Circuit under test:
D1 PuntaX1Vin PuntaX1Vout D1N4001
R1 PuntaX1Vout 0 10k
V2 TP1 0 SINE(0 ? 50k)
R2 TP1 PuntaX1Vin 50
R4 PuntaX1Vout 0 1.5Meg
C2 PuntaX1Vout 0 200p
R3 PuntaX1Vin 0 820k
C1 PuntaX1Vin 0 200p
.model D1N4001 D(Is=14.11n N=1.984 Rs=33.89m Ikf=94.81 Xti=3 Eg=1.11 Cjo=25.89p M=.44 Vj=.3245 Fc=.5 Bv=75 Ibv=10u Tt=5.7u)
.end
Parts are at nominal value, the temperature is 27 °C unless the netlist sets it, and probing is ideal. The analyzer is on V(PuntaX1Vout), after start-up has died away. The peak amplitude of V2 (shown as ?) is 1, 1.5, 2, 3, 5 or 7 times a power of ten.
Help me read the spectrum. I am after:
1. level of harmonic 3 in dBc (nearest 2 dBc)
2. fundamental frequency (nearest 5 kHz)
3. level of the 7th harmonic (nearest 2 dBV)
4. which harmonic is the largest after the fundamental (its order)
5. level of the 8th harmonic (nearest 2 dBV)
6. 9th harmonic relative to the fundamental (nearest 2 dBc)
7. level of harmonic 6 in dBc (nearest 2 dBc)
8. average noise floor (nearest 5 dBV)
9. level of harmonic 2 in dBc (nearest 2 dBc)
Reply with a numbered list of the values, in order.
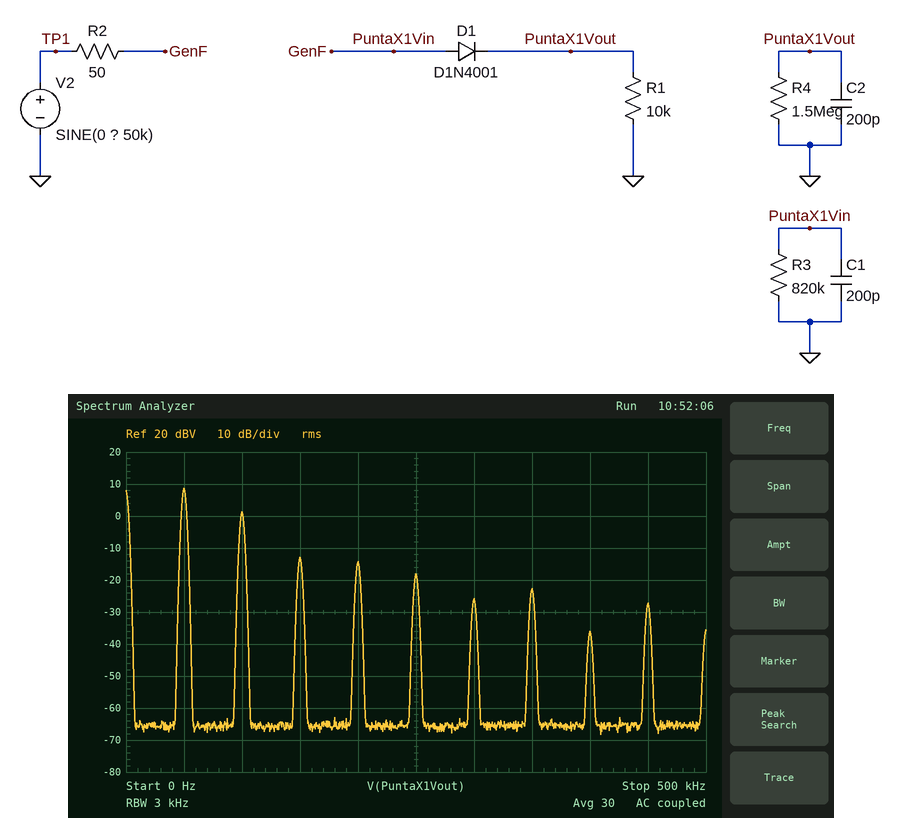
1. -22 dBc
2. 50 kHz
3. -22 dBV
4. 2
5. -36 dBV
6. -36 dBc
7. -34 dBc
8. -65 dBV
9. -8 dBc
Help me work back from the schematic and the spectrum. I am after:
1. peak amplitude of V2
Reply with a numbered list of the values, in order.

1. 7 V
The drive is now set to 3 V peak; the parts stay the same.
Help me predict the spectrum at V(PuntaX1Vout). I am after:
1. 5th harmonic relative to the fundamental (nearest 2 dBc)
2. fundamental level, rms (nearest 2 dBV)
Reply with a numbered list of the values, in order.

1. -30 dBc
2. 0 dBV
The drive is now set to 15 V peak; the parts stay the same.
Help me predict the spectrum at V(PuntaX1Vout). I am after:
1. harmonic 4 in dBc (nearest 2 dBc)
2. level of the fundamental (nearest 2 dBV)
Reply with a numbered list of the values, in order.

1. -24 dBc
2. 16 dBV
